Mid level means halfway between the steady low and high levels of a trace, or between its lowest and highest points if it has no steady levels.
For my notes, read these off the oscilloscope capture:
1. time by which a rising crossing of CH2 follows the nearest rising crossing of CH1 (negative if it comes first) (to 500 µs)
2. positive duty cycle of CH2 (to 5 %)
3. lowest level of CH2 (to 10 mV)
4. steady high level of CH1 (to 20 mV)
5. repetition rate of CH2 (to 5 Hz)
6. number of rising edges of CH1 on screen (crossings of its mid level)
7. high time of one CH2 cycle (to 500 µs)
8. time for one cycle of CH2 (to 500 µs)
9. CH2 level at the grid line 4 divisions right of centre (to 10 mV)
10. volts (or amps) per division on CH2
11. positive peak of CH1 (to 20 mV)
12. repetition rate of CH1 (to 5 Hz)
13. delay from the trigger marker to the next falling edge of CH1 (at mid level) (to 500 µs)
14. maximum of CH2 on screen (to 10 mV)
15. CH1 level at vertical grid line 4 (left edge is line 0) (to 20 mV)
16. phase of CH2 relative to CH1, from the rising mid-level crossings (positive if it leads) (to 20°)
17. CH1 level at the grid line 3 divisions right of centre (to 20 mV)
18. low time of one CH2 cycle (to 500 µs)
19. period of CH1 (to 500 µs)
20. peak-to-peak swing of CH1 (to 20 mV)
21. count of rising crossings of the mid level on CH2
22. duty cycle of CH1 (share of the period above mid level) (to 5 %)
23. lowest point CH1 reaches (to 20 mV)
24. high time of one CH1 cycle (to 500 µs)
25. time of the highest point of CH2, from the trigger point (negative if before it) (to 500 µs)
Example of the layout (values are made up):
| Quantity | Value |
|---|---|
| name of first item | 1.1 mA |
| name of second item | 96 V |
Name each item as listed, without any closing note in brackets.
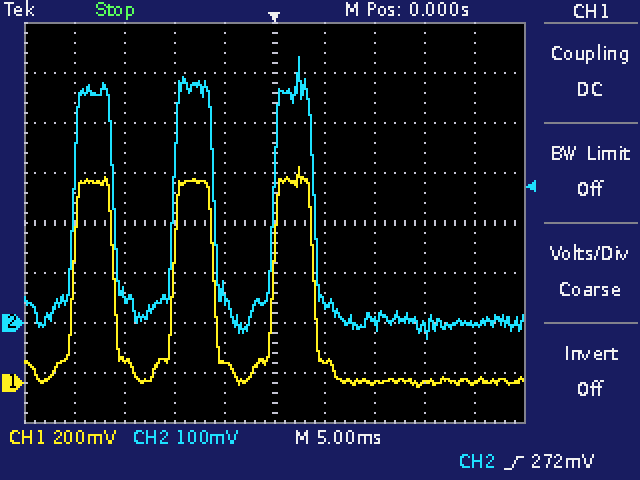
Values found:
| Quantity | Value |
|---|---|
| time by which a rising crossing of CH2 follows the nearest rising crossing of CH1 (negative if it comes first) | 0.0 ms |
| positive duty cycle of CH2 | 40 % |
| lowest level of CH2 | -30 mV |
| steady high level of CH1 | 800 mV |
| repetition rate of CH2 | 100 Hz |
| number of rising edges of CH1 on screen | 3 |
| high time of one CH2 cycle | 4.0 ms |
| time for one cycle of CH2 | 10.0 ms |
| CH2 level at the grid line 4 divisions right of centre | 0 mV |
| volts (or amps) per division on CH2 | 100 mV |
| positive peak of CH1 | 860 mV |
| repetition rate of CH1 | 100 Hz |
| delay from the trigger marker to the next falling edge of CH1 (at mid level) | 4.0 ms |
| maximum of CH2 on screen | 530 mV |
| CH1 level at vertical grid line 4 (left edge is line 0) | 80 mV |
| phase of CH2 relative to CH1, from the rising mid-level crossings (positive if it leads) | 0° |
| CH1 level at the grid line 3 divisions right of centre | 0 mV |
| low time of one CH2 cycle | 6.0 ms |
| period of CH1 | 10.0 ms |
| peak-to-peak swing of CH1 | 880 mV |
| count of rising crossings of the mid level on CH2 | 3 |
| duty cycle of CH1 (share of the period above mid level) | 40 % |
| lowest point CH1 reaches | -20 mV |
| high time of one CH1 cycle | 4.0 ms |
| time of the highest point of CH2, from the trigger point (negative if before it) | +2.5 ms |
